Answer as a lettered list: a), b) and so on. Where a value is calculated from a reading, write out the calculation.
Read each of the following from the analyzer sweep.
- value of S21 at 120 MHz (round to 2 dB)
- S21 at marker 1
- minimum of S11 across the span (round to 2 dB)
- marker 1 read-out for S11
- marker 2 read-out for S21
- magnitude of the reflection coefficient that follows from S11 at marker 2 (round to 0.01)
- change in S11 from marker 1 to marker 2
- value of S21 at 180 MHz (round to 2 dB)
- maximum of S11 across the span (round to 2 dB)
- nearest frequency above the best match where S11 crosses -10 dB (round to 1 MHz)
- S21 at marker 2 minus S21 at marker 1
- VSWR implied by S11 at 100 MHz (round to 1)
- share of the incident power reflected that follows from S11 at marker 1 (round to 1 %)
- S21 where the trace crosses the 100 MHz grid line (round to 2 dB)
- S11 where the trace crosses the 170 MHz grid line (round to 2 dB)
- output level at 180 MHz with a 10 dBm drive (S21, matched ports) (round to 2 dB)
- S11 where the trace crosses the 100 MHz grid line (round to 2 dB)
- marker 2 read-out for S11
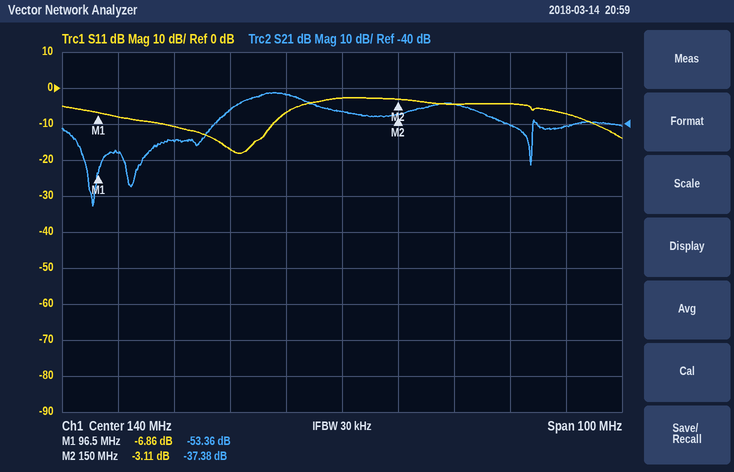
a) -36 dB
b) -53.36 dB
c) -18 dB
d) -6.86 dB
e) -37.38 dB
f) 10^(-3.11/20) ≈ 0.70
g) -3.11 − (-6.86) = 3.75 dB
h) -40 dB
i) -2 dB
j) 128 MHz
k) -37.38 − (-53.36) = 15.98 dB
l) |Γ| = 10^(-8/20) = 0.3981; VSWR = (1 + 0.3981)/(1 − 0.3981) ≈ 2
m) 10^(-6.86/10) ≈ 21 %
n) -48 dB
o) -4 dB
p) 10 dBm + (-40 dB) = -30 dBm
q) -8 dB
r) -3.11 dB
